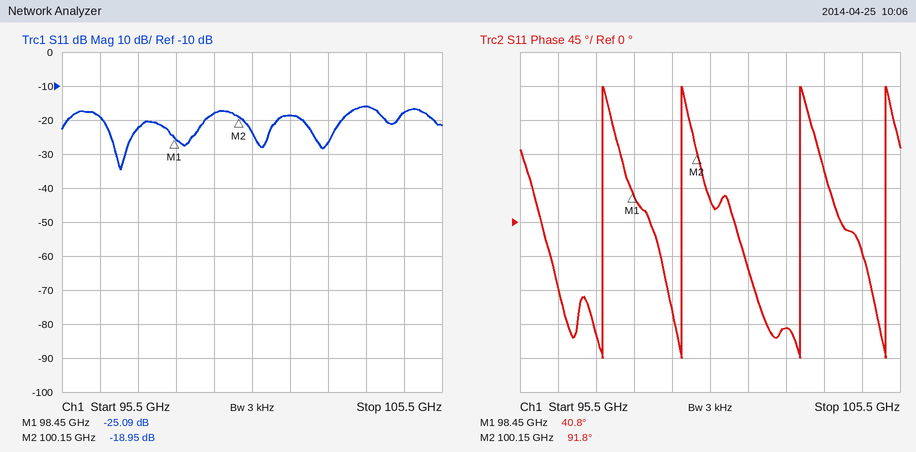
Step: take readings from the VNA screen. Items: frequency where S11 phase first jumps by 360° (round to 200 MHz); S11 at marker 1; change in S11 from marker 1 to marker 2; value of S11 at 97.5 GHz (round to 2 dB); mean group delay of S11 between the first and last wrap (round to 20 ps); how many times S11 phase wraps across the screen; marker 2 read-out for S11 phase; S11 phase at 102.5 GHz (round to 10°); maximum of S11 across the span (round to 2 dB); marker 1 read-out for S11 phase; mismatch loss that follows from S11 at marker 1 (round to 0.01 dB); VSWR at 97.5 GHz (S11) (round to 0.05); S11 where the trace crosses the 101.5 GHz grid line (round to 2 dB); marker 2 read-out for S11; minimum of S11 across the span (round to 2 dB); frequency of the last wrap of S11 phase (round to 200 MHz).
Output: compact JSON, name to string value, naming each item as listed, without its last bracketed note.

{"frequency where S11 phase first jumps by 360°": "97.6 GHz", "S11 at marker 1": "-25.09 dB", "change in S11 from marker 1 to marker 2": "6.14 dB", "value of S11 at 97.5 GHz": "-22 dB", "mean group delay of S11 between the first and last wrap": "400 ps", "how many times S11 phase wraps across the screen": "4", "marker 2 read-out for S11 phase": "91.8°", "S11 phase at 102.5 GHz": "-140°", "maximum of S11 across the span": "-16 dB", "marker 1 read-out for S11 phase": "40.8°", "mismatch loss that follows from S11 at marker 1": "0.01 dB", "VSWR at 97.5 GHz (S11)": "1.15", "S11 where the trace crosses the 101.5 GHz grid line": "-18 dB", "marker 2 read-out for S11": "-18.95 dB", "minimum of S11 across the span": "-34 dB", "frequency of the last wrap of S11 phase": "105.2 GHz"}
